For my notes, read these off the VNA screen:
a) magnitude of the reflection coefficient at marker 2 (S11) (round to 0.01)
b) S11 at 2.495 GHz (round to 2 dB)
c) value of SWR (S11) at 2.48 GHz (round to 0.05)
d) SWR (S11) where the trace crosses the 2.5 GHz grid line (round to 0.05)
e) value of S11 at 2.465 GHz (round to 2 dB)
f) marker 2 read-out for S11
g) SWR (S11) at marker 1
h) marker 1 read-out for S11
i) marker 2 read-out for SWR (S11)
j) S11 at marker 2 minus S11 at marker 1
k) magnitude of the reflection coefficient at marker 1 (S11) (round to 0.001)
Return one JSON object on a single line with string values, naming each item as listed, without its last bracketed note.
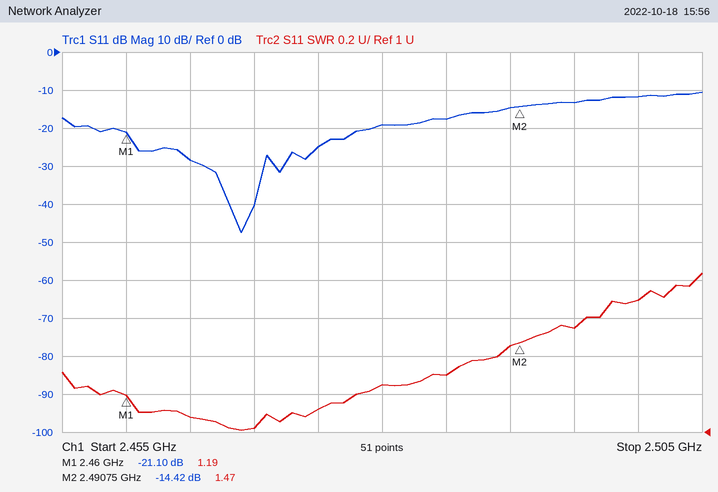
{"magnitude of the reflection coefficient at marker 2 (S11)": "0.19", "S11 at 2.495 GHz": "-14 dB", "value of SWR (S11) at 2.48 GHz": "1.25", "SWR (S11) where the trace crosses the 2.5 GHz grid line": "1.70", "value of S11 at 2.465 GHz": "-28 dB", "marker 2 read-out for S11": "-14.42 dB", "SWR (S11) at marker 1": "1.19", "marker 1 read-out for S11": "-21.10 dB", "marker 2 read-out for SWR": "1.47", "S11 at marker 2 minus S11 at marker 1": "6.68 dB", "magnitude of the reflection coefficient at marker 1 (S11)": "0.088"}
